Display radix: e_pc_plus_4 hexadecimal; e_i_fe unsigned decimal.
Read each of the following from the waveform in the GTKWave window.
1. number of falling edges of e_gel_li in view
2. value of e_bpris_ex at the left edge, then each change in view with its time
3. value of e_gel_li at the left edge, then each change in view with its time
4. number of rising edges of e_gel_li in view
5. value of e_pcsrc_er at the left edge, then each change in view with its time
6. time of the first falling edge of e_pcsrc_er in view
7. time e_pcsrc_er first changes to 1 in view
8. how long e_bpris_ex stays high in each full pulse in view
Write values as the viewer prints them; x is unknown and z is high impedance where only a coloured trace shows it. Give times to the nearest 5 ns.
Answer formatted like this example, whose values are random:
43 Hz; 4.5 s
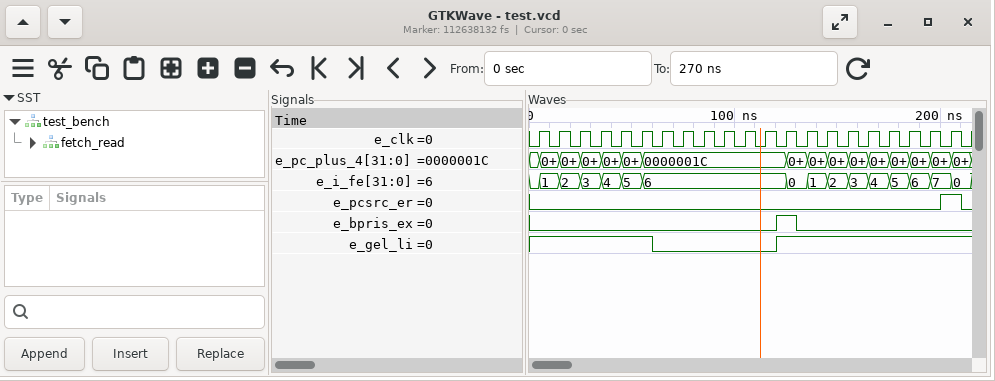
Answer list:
1; 0, 1 at 120 ns, 0 at 130 ns; 1, 0 at 60 ns, 1 at 120 ns; 1; 0, 1 at 200 ns, 0 at 210 ns; 210 ns; 200 ns; 10 ns
